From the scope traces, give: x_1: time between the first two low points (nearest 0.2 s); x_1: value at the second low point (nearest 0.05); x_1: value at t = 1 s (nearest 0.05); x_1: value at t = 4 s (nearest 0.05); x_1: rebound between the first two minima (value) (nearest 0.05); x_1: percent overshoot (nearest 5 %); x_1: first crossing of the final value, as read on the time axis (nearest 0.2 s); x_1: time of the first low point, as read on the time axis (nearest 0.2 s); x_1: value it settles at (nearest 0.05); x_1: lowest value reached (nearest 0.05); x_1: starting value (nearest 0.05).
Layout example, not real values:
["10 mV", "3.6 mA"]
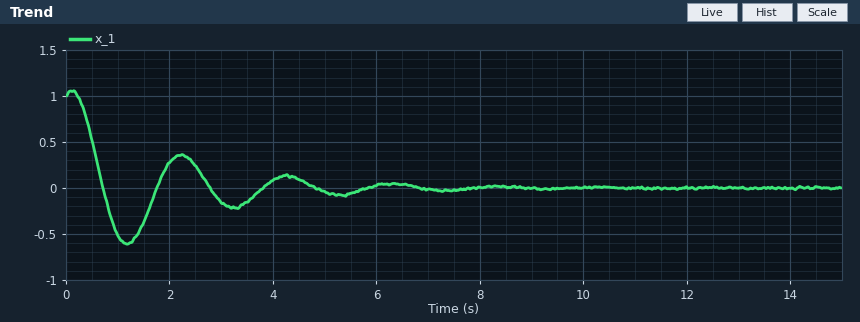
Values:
["2.0 s", "-0.20", "-0.50", "0.10", "0.35", "60 %", "0.8 s", "1.2 s", "0.00", "-0.60", "1.00"]
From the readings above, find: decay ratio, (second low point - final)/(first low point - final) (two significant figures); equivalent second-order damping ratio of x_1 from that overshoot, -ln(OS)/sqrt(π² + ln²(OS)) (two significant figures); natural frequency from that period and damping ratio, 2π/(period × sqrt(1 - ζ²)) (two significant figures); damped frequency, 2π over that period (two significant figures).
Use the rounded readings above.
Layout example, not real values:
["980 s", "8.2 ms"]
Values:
["0.33", "0.16", "3.2 rad/s", "3.1 rad/s"]
